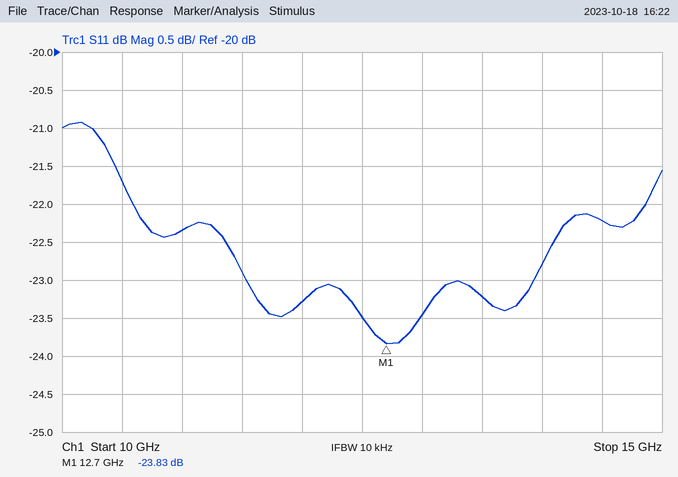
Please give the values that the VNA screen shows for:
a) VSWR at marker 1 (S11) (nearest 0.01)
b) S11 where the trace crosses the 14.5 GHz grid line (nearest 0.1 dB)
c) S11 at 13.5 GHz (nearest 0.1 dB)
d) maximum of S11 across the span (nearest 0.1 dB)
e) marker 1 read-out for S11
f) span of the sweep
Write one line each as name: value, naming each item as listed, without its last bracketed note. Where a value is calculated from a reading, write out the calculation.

VSWR at marker 1 (S11): (1 + 0.0643)/(1 − 0.0643) ≈ 1.14
S11 where the trace crosses the 14.5 GHz grid line: -22.2 dB
S11 at 13.5 GHz: -23.2 dB
maximum of S11 across the span: -20.9 dB
marker 1 read-out for S11: -23.83 dB
span of the sweep: 5 GHz
